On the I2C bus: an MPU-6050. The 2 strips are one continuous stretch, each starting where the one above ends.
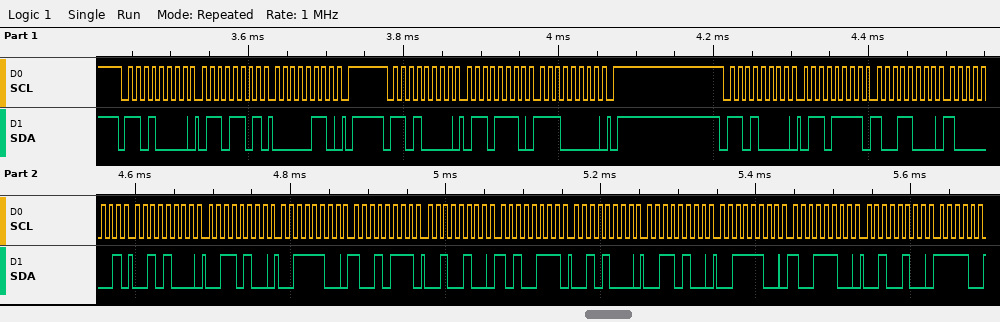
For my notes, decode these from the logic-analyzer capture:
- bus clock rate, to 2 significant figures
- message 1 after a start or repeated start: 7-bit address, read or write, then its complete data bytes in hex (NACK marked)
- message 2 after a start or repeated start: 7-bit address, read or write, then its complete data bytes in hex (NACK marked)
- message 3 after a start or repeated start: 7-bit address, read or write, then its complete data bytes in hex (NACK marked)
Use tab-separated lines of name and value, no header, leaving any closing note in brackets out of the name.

bus clock rate, to 2 significant figures	100 kHz
message 1 after a start or repeated start: 7-bit address, read or write, then its complete data bytes in hex	0x68 write: 6D 06
message 2 after a start or repeated start: 7-bit address, read or write, then its complete data bytes in hex	0x68 write: 6E E0
message 3 after a start or repeated start: 7-bit address, read or write, then its complete data bytes in hex	0x68 write: 6F 98 81 28 34 3C 97 24 A7 28 34 3C 9C 24
